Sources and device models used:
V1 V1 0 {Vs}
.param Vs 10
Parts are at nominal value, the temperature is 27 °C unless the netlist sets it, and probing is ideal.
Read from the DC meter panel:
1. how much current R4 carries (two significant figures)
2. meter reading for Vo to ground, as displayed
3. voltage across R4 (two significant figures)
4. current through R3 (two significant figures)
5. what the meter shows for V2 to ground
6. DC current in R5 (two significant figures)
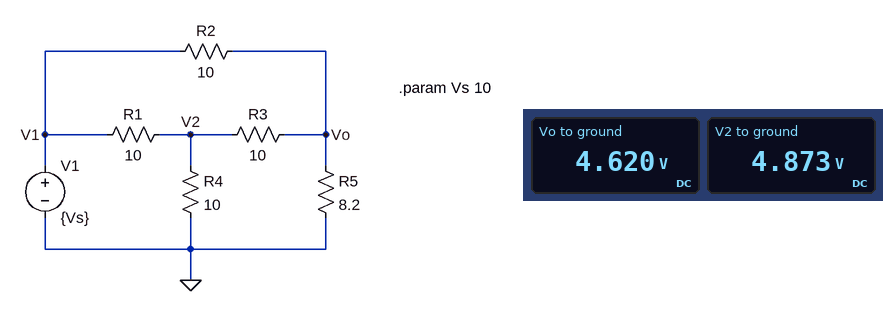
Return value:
490 mA
4.620 V
4.9 V
25 mA
4.873 V
560 mA
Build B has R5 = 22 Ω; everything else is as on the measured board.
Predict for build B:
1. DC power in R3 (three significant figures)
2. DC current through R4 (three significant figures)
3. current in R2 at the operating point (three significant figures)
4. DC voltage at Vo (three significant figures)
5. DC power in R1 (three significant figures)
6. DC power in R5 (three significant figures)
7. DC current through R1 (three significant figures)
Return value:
73.5 mW
543 mA
371 mA
6.29 V
2.09 W
1.80 W
457 mA
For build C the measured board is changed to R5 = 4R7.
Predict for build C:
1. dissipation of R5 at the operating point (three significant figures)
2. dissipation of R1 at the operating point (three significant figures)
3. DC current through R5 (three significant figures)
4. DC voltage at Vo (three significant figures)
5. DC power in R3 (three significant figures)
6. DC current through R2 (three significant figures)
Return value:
2.63 W
3.02 W
748 mA
3.51 V
98.1 mW
649 mA
